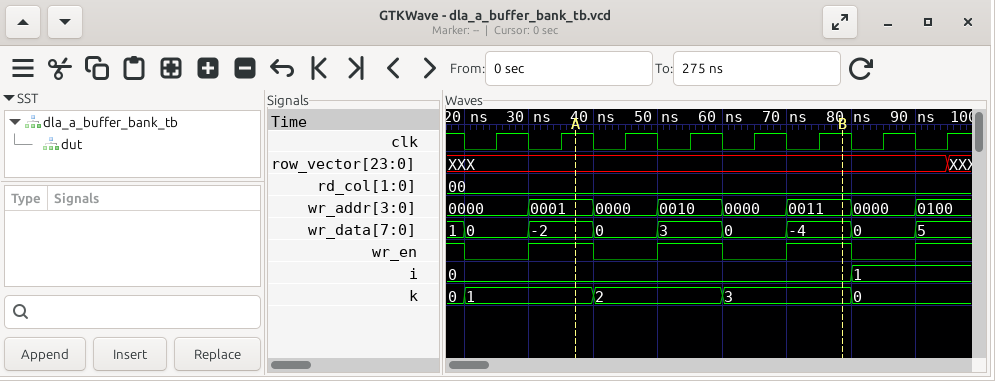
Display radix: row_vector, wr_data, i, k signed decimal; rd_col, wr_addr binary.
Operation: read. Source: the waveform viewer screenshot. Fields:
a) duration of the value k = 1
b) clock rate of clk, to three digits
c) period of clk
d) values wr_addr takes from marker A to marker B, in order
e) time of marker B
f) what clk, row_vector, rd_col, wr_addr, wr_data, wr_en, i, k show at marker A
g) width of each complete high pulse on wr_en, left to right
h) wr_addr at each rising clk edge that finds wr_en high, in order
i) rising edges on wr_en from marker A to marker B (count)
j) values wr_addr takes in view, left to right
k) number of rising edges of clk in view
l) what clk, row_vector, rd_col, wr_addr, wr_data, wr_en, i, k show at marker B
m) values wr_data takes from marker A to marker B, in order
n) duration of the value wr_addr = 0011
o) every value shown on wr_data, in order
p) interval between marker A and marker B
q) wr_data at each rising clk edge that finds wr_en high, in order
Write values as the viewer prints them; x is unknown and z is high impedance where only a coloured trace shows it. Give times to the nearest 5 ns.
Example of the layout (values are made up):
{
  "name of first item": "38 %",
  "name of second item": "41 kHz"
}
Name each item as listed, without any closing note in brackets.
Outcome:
{
  "duration of the value k = 1": "20 ns",
  "clock rate of clk, to three digits": "100 MHz",
  "period of clk": "10 ns",
  "values wr_addr takes from marker A to marker B, in order": "0001, 0000, 0010, 0000, 0011",
  "time of marker B": "80 ns",
  "what clk, row_vector, rd_col, wr_addr, wr_data, wr_en, i, k show at marker A": "clk=1, row_vector=XXX, rd_col=00, wr_addr=0001, wr_data=-2, wr_en=1, i=0, k=1",
  "width of each complete high pulse on wr_en, left to right": "10 ns, 10 ns, 10 ns",
  "wr_addr at each rising clk edge that finds wr_en high, in order": "0001, 0010, 0011, 0100",
  "rising edges on wr_en from marker A to marker B": "2",
  "values wr_addr takes in view, left to right": "0000, 0001, 0000, 0010, 0000, 0011, 0000, 0100",
  "number of rising edges of clk in view": "8",
  "what clk, row_vector, rd_col, wr_addr, wr_data, wr_en, i, k show at marker B": "clk=1, row_vector=XXX, rd_col=00, wr_addr=0011, wr_data=-4, wr_en=1, i=0, k=3",
  "values wr_data takes from marker A to marker B, in order": "-2, 0, 3, 0, -4",
  "duration of the value wr_addr = 0011": "10 ns",
  "every value shown on wr_data, in order": "1, 0, -2, 0, 3, 0, -4, 0, 5",
  "interval between marker A and marker B": "40 ns",
  "wr_data at each rising clk edge that finds wr_en high, in order": "-2, 3, -4, 5"
}
